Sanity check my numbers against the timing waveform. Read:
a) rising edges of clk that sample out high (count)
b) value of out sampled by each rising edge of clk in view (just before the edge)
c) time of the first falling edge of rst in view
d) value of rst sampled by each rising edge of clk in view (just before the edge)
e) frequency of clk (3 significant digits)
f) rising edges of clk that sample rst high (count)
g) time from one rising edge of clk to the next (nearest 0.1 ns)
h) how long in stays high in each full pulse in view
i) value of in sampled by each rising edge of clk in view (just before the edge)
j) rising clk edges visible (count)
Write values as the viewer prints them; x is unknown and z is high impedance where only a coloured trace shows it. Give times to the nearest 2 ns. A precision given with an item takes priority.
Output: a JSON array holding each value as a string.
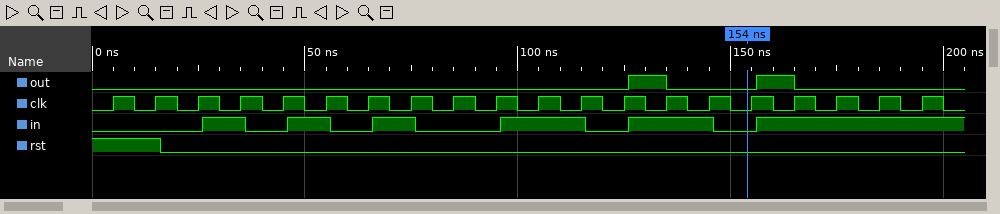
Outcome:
["2", "0 0 0 0 0 0 0 0 0 0 0 0 0 1 0 0 1 0 0 0", "16 ns", "1 1 0 0 0 0 0 0 0 0 0 0 0 0 0 0 0 0 0 0", "100 MHz", "2", "10 ns", "10 ns, 10 ns, 10 ns, 20 ns, 20 ns", "0 0 0 1 0 1 0 1 0 0 1 1 0 1 1 0 1 1 1 1", "20"]
